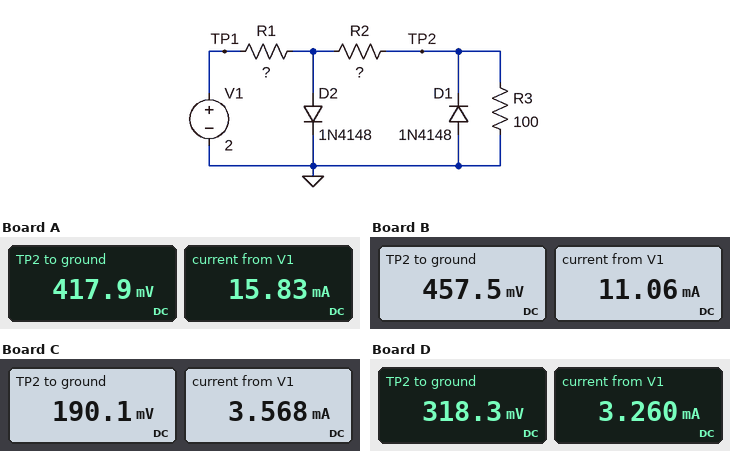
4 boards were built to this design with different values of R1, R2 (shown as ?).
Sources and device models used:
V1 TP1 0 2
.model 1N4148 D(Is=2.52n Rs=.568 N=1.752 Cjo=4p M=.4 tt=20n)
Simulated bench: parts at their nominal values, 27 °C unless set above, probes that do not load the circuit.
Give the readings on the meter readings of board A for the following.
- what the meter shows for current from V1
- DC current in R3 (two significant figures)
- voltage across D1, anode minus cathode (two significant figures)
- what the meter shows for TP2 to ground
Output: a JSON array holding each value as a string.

["15.83 mA", "4.2 mA", "-420 mV", "417.9 mV"]
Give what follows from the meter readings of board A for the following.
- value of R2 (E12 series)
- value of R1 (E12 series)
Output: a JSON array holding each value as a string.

["68 Ω", "82 Ω"]
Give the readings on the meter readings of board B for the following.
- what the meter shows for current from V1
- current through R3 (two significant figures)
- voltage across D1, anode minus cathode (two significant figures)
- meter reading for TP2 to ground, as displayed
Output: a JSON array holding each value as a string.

["11.06 mA", "4.6 mA", "-460 mV", "457.5 mV"]
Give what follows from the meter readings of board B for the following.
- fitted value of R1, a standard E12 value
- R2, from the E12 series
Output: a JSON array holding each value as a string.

["120 Ω", "47 Ω"]
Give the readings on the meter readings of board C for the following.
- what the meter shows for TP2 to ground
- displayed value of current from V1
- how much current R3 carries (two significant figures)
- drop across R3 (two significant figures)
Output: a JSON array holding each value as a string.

["190.1 mV", "3.568 mA", "1.9 mA", "190 mV"]
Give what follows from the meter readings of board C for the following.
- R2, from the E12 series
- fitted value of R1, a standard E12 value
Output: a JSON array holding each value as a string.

["220 Ω", "390 Ω"]
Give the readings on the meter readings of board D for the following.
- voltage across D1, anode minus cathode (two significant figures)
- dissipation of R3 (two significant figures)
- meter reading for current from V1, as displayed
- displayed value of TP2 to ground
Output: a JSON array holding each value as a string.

["-320 mV", "1.0 mW", "3.260 mA", "318.3 mV"]
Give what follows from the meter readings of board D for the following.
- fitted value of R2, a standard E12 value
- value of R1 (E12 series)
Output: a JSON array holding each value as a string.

["47 Ω", "470 Ω"]
